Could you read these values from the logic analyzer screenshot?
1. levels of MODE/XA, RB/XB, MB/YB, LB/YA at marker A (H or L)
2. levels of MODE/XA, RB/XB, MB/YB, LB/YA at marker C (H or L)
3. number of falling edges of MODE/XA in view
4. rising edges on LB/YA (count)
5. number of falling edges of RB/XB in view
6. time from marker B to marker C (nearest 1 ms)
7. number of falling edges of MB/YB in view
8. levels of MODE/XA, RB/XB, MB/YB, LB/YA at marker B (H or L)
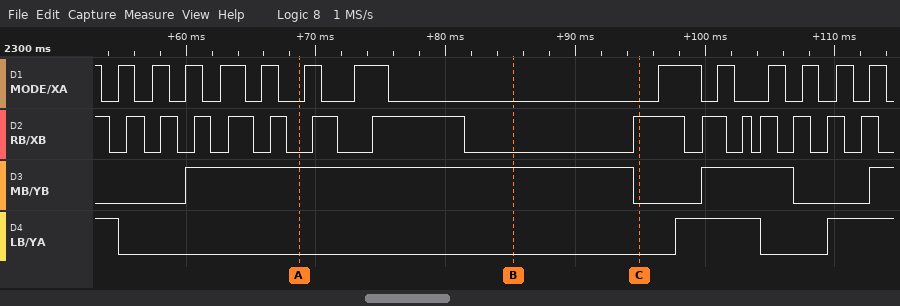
MODE/XA=L, RB/XB=L, MB/YB=H, LB/YA=L
MODE/XA=L, RB/XB=H, MB/YB=L, LB/YA=L
14
2
15
10 ms
2
MODE/XA=L, RB/XB=L, MB/YB=H, LB/YA=L
